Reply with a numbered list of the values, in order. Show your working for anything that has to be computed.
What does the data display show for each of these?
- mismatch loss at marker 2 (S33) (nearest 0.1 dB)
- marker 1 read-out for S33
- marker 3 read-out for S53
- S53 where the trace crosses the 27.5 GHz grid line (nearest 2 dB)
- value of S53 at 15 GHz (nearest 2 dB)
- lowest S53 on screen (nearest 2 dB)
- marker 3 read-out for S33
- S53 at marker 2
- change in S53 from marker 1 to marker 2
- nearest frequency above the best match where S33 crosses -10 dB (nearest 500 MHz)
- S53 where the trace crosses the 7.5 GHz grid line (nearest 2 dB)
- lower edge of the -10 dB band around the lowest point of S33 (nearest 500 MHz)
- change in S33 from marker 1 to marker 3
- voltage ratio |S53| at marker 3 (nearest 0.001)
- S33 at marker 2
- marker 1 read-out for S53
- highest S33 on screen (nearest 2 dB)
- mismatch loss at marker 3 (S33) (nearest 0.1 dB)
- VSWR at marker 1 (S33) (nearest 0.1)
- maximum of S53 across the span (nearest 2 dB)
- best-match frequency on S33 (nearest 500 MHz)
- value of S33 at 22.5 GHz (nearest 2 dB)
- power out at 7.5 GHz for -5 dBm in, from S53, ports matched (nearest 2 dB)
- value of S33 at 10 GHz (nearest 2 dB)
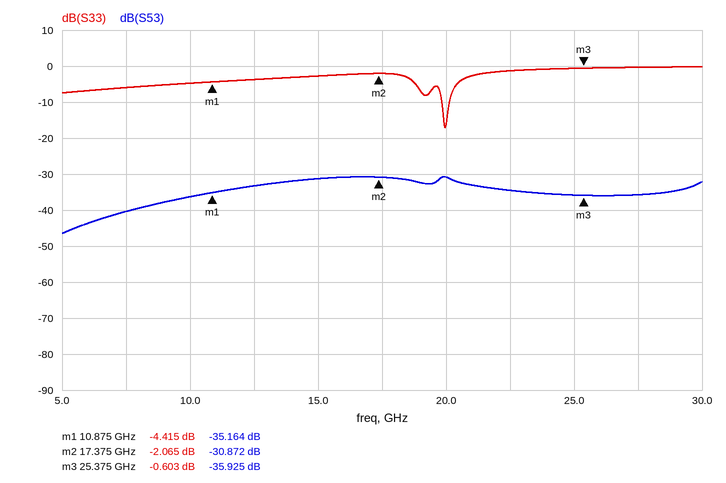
1. −10 log10(1 − 10^(-2.065/10)) ≈ 4.2 dB
2. -4.415 dB
3. -35.925 dB
4. -36 dB
5. -32 dB
6. -46 dB
7. -0.603 dB
8. -30.872 dB
9. -30.872 − (-35.164) = 4.292 dB
10. 20.0 GHz
11. -40 dB
12. 20.0 GHz
13. -0.603 − (-4.415) = 3.812 dB
14. 10^(-35.925/20) ≈ 0.016
15. -2.065 dB
16. -35.164 dB
17. 0 dB
18. −10 log10(1 − 10^(-0.603/10)) ≈ 8.9 dB
19. (1 + 0.6015)/(1 − 0.6015) ≈ 4.0
20. -30 dB
21. 20.0 GHz
22. -2 dB
23. -5 dBm + (-40 dB) = -46 dBm
24. -4 dB
